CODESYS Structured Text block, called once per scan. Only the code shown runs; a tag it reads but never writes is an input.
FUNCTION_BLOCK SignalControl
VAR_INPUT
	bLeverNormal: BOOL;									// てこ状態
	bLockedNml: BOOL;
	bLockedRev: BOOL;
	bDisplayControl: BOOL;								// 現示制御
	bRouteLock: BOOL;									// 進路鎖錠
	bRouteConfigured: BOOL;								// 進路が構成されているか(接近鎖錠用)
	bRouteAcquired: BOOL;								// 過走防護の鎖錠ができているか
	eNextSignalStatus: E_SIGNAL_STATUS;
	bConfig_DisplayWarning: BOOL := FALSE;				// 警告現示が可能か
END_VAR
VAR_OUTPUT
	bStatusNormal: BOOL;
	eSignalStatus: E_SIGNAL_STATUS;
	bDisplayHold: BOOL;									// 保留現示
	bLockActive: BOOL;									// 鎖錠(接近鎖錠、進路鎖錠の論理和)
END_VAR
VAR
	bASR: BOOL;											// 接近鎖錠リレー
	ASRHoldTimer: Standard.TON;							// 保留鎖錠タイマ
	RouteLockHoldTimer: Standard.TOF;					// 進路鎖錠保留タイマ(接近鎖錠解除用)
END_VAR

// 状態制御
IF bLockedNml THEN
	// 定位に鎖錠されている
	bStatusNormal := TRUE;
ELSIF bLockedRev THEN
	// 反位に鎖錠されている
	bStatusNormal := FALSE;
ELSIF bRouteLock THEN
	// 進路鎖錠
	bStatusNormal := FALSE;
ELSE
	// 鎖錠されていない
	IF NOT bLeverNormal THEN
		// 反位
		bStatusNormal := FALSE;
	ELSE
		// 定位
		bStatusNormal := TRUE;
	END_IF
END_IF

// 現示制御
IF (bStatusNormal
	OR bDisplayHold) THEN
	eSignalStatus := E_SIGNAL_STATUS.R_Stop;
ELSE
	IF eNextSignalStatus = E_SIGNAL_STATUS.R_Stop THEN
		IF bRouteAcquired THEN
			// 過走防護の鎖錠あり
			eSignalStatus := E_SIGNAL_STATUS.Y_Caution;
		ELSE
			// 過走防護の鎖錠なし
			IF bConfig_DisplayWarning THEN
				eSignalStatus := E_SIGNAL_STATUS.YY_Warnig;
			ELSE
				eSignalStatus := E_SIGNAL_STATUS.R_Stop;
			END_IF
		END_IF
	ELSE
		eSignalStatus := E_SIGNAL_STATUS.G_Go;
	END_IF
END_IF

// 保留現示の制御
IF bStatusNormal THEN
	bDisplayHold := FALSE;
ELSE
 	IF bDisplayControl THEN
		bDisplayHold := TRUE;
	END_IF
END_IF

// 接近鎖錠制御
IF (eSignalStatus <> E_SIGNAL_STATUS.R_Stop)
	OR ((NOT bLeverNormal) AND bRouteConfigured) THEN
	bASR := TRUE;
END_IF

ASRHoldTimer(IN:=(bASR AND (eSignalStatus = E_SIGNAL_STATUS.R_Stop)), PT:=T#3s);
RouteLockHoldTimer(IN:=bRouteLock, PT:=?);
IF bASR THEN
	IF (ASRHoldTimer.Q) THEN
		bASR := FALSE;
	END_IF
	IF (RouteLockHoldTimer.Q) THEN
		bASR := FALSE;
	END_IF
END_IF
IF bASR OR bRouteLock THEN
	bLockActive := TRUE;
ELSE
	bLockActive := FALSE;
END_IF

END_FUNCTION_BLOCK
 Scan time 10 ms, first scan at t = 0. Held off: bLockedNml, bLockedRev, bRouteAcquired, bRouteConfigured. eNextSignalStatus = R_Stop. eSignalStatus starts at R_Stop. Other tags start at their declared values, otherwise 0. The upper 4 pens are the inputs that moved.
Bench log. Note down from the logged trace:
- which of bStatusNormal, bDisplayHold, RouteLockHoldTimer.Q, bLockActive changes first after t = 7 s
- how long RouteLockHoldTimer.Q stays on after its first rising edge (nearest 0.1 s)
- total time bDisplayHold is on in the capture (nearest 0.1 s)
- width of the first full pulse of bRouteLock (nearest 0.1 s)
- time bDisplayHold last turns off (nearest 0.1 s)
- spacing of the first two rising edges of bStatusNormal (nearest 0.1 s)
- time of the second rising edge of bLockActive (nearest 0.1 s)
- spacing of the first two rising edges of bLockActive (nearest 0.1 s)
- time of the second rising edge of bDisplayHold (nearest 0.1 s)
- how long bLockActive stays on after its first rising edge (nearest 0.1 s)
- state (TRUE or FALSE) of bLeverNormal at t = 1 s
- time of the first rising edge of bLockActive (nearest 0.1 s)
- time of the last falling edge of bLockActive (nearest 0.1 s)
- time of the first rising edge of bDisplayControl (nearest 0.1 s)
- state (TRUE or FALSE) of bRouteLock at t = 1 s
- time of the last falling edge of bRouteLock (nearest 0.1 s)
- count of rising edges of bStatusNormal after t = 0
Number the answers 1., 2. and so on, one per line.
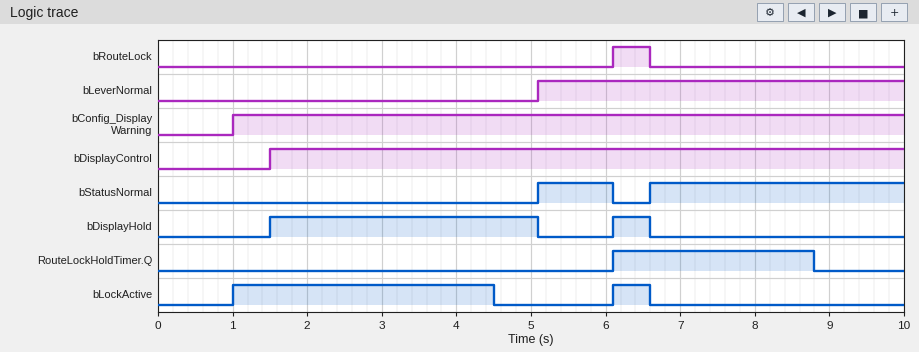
1. RouteLockHoldTimer.Q
2. 2.7 s
3. 4.1 s
4. 0.5 s
5. 6.6 s
6. 1.5 s
7. 6.1 s
8. 5.1 s
9. 6.1 s
10. 3.5 s
11. FALSE
12. 1.0 s
13. 6.6 s
14. 1.5 s
15. FALSE
16. 6.6 s
17. 2
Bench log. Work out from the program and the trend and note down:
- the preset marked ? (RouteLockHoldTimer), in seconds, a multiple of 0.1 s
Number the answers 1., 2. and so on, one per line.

1. 2.2 s
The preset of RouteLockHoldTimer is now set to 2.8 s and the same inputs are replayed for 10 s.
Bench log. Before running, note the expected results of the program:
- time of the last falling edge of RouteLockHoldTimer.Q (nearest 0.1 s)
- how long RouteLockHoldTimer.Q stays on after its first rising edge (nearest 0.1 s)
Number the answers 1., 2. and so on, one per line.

1. 9.4 s
2. 3.3 s
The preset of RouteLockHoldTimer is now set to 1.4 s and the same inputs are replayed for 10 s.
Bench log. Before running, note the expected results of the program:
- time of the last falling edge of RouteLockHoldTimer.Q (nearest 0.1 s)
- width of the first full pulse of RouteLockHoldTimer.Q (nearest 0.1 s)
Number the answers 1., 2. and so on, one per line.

1. 8.0 s
2. 1.9 s
